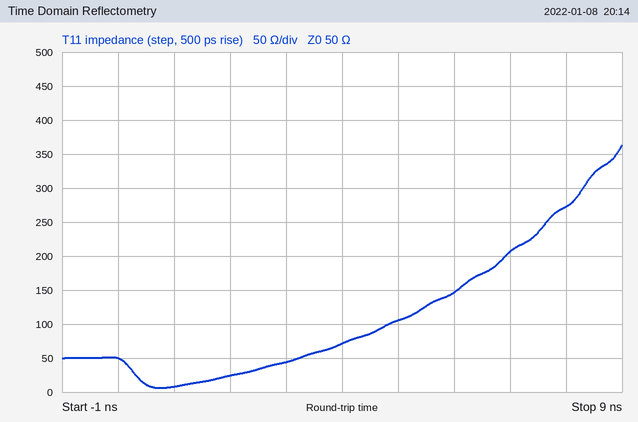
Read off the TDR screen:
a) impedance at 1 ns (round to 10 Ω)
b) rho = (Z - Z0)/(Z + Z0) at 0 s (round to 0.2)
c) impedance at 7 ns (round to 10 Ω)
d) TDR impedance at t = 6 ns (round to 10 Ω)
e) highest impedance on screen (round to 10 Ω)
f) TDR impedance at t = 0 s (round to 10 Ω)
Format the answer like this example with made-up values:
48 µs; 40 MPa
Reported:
10 Ω; 0.0; 210 Ω; 150 Ω; 360 Ω; 50 Ω
